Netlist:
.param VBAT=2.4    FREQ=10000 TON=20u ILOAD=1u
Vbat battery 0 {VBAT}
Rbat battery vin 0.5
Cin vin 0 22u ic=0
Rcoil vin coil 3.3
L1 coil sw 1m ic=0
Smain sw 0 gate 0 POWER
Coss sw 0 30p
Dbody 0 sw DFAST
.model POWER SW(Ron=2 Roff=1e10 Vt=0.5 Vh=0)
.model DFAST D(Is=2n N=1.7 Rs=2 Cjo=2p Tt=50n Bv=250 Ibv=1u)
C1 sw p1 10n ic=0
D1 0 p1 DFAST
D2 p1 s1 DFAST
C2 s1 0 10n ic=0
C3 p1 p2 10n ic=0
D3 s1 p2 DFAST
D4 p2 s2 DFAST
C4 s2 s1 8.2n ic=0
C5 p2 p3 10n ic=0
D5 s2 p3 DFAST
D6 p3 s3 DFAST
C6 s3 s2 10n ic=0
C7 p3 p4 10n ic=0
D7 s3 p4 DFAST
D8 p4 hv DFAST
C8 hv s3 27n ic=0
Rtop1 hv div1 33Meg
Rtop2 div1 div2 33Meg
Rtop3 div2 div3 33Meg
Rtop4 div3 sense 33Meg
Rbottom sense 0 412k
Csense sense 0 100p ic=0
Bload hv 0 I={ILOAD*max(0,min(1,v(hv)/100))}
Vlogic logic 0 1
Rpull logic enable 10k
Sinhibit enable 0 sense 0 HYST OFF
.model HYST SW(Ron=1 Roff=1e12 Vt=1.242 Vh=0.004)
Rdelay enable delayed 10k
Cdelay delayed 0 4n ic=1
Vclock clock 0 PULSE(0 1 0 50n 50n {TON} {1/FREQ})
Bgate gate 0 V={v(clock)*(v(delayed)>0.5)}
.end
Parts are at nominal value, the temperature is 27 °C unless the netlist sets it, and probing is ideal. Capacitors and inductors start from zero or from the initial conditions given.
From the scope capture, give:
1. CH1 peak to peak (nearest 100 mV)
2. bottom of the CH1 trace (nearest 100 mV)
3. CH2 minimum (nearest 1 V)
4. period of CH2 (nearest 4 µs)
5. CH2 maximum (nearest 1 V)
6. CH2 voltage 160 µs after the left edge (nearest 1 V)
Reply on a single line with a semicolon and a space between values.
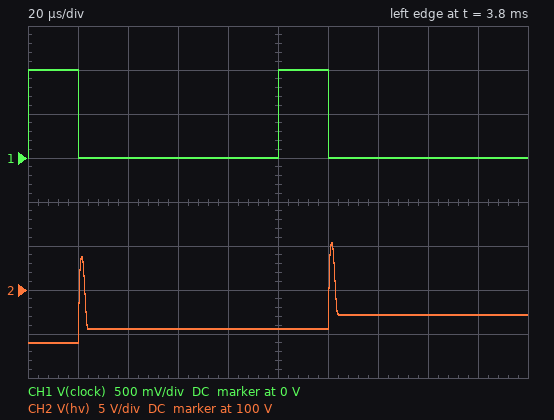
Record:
1.0 V; 0 V; 94 V; 100 µs; 105 V; 97 V
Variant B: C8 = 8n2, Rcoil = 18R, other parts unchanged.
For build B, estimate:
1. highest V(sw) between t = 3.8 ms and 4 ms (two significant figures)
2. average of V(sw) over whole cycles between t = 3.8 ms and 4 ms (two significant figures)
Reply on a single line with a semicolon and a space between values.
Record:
35 V; 2.3 V
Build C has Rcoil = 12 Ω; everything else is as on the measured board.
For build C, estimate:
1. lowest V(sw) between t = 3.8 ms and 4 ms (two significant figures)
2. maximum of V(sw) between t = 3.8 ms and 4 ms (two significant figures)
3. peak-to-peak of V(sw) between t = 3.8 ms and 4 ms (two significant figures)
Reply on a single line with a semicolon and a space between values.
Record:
-720 mV; 35 V; 36 V
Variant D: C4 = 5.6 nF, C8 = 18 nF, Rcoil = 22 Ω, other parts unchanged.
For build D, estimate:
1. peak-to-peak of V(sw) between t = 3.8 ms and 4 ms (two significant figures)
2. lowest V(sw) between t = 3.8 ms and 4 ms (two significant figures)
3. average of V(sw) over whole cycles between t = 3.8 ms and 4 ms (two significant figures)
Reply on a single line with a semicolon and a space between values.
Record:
34 V; -700 mV; 2.3 V
